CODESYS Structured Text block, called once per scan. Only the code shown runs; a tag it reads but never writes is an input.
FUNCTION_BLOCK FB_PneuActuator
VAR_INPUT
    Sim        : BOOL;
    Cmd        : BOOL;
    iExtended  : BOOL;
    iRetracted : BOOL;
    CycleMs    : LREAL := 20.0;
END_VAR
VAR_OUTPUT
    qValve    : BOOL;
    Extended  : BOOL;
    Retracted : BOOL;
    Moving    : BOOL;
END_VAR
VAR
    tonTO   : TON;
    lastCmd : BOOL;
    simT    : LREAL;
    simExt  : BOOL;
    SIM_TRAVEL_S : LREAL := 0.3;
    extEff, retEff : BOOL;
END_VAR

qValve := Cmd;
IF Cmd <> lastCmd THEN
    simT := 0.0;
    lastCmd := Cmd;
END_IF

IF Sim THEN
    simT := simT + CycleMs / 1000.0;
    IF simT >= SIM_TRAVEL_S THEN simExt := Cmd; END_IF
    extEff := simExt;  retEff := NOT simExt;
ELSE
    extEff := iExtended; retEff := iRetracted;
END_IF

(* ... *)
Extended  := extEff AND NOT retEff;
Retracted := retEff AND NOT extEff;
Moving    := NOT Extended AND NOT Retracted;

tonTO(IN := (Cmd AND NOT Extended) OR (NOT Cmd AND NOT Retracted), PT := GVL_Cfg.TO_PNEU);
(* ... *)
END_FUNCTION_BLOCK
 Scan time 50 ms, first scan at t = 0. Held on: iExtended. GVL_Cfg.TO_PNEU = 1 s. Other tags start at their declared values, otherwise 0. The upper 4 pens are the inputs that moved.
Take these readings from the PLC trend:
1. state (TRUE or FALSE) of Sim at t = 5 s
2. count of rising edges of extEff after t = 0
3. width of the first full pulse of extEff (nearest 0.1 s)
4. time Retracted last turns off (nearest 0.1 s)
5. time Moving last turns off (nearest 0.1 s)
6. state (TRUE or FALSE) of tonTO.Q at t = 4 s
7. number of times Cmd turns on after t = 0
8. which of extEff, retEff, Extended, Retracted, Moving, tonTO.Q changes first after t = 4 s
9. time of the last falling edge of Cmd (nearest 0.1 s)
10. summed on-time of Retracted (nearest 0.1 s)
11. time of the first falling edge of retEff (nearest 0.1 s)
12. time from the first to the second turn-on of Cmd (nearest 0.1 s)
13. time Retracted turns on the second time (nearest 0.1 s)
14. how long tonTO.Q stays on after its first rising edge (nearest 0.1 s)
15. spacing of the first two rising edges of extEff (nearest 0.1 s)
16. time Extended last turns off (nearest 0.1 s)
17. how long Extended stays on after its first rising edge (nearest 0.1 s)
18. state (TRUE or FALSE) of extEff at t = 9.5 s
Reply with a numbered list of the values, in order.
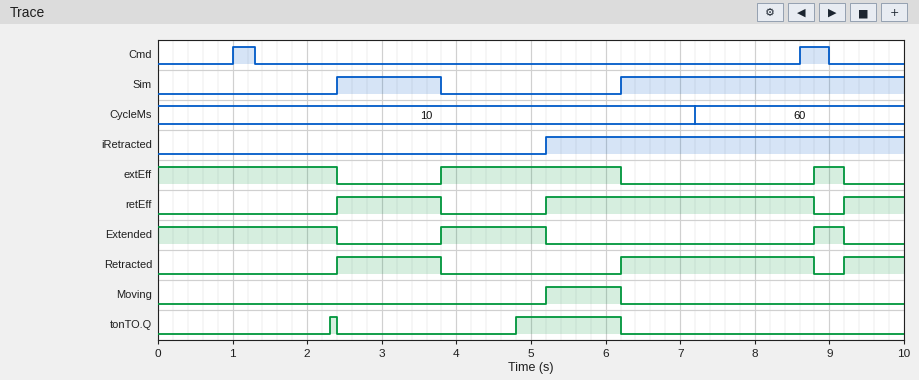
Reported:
1. FALSE
2. 2
3. 2.4 s
4. 8.8 s
5. 6.2 s
6. FALSE
7. 2
8. tonTO.Q
9. 9.0 s
10. 4.8 s
11. 3.8 s
12. 7.6 s
13. 6.2 s
14. 0.1 s
15. 5.0 s
16. 9.2 s
17. 1.4 s
18. FALSE
